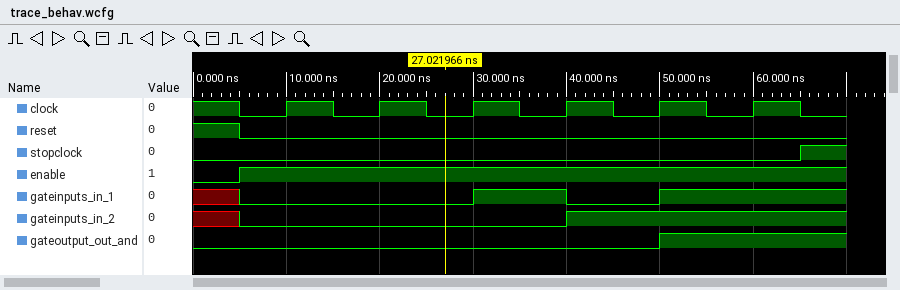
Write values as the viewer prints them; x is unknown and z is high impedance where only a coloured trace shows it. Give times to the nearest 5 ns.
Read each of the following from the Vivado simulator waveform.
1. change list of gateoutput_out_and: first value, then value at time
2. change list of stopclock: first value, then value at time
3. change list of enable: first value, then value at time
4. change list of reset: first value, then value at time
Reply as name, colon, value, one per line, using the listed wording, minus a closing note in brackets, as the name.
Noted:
change list of gateoutput_out_and: first value, then value at time: 0, 1 at 50 ns
change list of stopclock: first value, then value at time: 0, 1 at 65 ns
change list of enable: first value, then value at time: 0, 1 at 5 ns
change list of reset: first value, then value at time: 1, 0 at 5 ns
